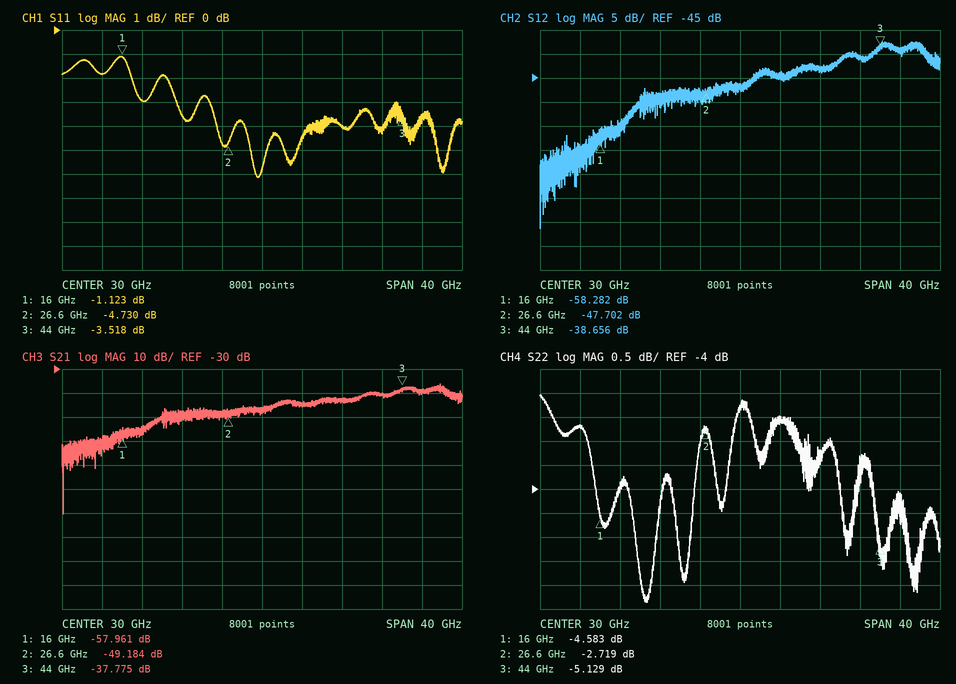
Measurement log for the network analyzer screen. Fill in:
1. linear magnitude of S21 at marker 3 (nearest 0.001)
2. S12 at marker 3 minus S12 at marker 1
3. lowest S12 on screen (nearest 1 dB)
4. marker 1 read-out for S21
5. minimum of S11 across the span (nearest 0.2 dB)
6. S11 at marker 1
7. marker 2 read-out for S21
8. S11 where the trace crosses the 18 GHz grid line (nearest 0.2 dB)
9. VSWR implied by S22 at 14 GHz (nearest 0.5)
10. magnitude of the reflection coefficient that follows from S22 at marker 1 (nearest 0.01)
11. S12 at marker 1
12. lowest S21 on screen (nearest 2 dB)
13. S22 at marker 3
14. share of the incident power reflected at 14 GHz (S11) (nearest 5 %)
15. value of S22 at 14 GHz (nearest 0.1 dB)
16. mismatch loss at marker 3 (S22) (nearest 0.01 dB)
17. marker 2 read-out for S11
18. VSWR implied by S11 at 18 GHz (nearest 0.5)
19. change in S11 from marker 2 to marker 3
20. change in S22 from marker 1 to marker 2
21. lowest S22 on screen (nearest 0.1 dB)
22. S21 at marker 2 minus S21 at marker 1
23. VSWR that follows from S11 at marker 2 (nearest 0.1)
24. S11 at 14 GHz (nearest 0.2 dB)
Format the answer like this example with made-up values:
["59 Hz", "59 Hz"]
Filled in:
["0.013", "19.626 dB", "-76 dB", "-57.961 dB", "-6.2 dB", "-1.123 dB", "-49.184 dB", "-3.0 dB", "6.5", "0.59", "-58.282 dB", "-90 dB", "-5.129 dB", "65 %", "-2.7 dB", "1.59 dB", "-4.730 dB", "6.0", "1.212 dB", "1.864 dB", "-6.4 dB", "8.777 dB", "3.8", "-1.8 dB"]
